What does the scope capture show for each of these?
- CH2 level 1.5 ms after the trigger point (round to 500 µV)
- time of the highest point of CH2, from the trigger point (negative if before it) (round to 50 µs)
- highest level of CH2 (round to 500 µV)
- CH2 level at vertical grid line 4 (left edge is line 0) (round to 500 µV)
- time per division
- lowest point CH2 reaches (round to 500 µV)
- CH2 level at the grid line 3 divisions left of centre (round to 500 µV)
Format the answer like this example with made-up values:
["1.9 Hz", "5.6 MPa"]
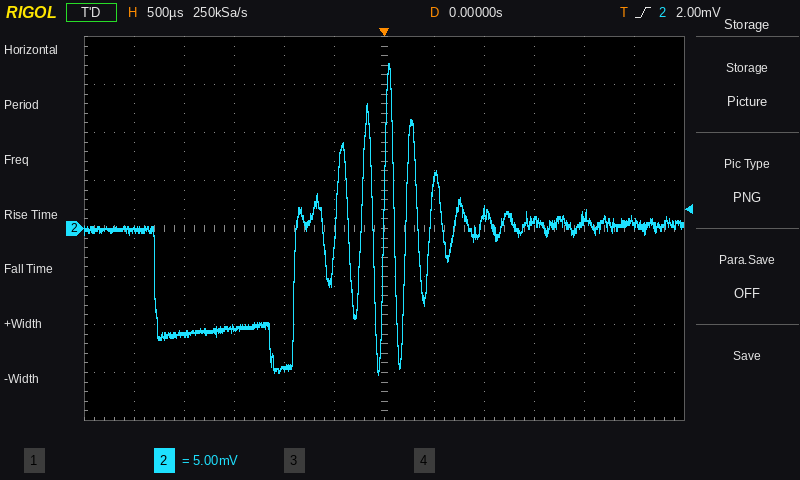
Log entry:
["500 µV", "+50 µs", "17.0 mV", "-14.5 mV", "500 µs", "-15.0 mV", "-10.5 mV"]
